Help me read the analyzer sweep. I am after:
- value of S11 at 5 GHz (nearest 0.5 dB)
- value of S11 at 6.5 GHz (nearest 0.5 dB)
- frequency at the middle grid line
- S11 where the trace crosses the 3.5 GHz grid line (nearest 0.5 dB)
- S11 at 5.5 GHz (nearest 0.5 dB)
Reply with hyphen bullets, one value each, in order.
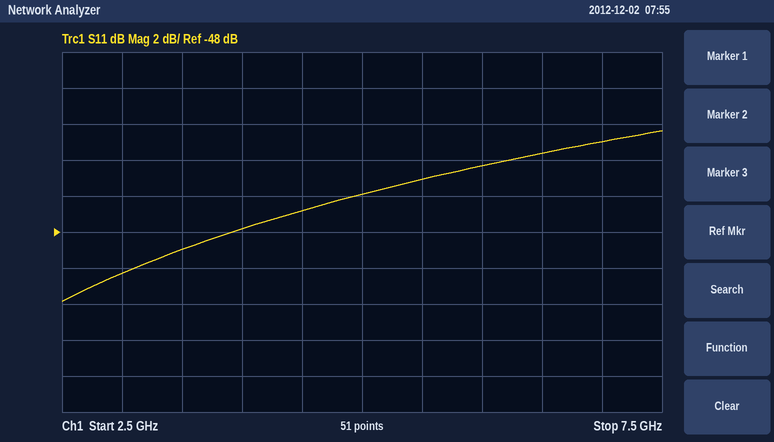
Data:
- -46.0 dB
- -43.5 dB
- 5 GHz
- -49.0 dB
- -45.0 dB
